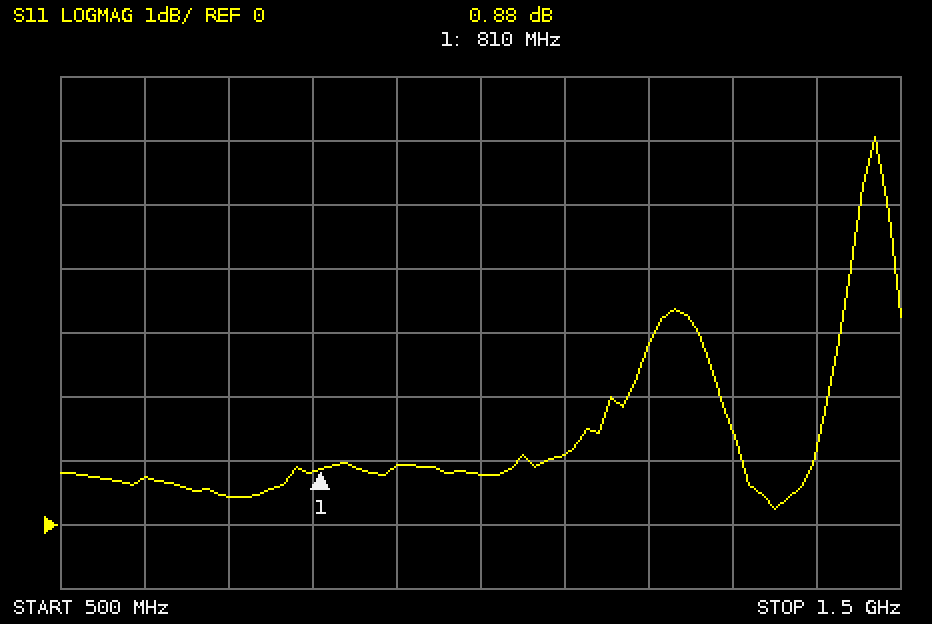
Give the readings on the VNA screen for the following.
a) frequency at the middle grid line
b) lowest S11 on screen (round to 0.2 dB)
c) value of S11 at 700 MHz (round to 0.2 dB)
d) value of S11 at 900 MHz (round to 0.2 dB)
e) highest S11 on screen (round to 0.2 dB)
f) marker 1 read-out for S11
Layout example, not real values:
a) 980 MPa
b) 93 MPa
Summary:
a) 1 GHz
b) 0.2 dB
c) 0.4 dB
d) 1.0 dB
e) 6.0 dB
f) 0.88 dB
